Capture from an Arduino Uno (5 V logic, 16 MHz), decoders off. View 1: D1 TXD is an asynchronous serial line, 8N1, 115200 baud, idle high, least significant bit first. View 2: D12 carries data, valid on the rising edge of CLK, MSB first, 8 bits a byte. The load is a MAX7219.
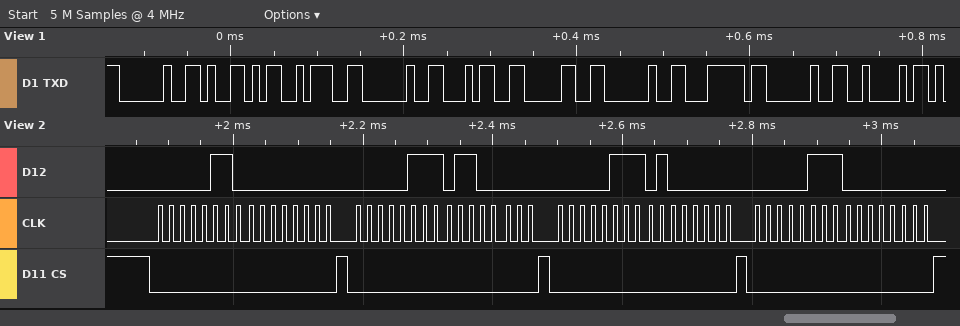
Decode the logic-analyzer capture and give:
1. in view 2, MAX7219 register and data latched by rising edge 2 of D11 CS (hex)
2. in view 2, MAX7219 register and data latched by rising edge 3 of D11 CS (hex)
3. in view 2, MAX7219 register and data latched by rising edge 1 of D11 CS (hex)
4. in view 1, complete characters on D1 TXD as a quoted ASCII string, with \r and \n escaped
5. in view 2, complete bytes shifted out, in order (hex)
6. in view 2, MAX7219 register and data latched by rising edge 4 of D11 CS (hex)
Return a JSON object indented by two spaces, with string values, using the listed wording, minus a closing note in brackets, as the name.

{
  "in view 2, MAX7219 register and data latched by rising edge 2 of D11 CS": "register 0x7, data 0x60",
  "in view 2, MAX7219 register and data latched by rising edge 3 of D11 CS": "register 0x7, data 0x40",
  "in view 2, MAX7219 register and data latched by rising edge 1 of D11 CS": "register 0x6, data 0x00",
  "in view 1, complete characters on D1 TXD as a quoted ASCII string, with \\r and \\n escaped": "\" Y: 40 | B\"",
  "in view 2, complete bytes shifted out, in order": "06 00 07 60 07 40 07 00",
  "in view 2, MAX7219 register and data latched by rising edge 4 of D11 CS": "register 0x7, data 0x00"
}
